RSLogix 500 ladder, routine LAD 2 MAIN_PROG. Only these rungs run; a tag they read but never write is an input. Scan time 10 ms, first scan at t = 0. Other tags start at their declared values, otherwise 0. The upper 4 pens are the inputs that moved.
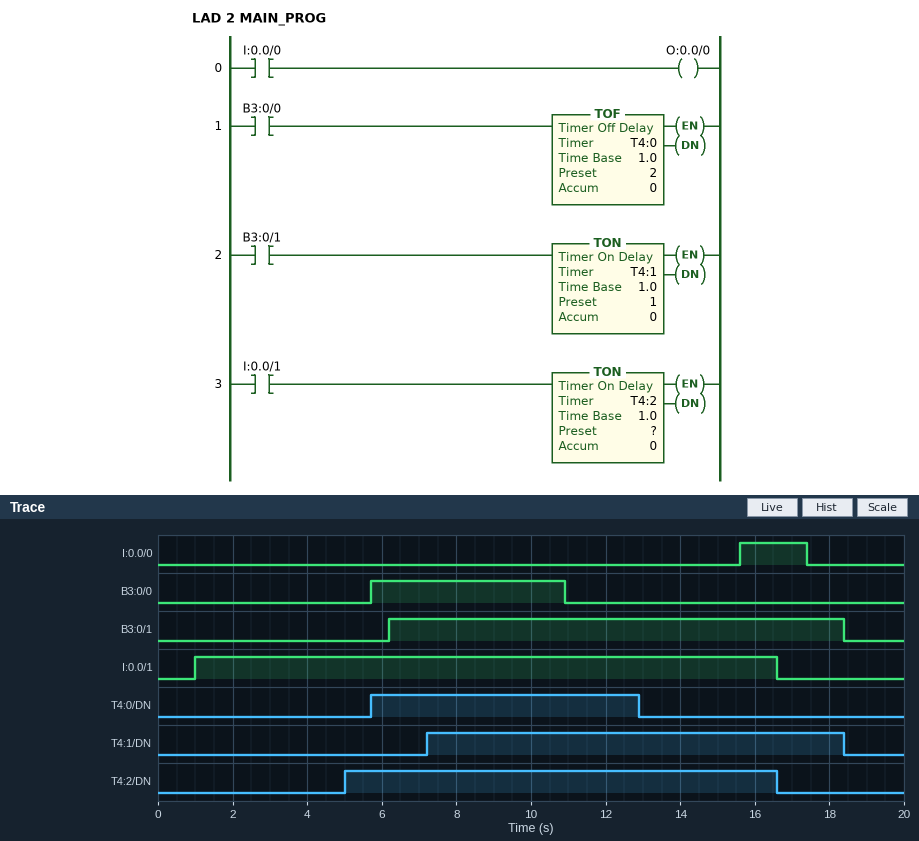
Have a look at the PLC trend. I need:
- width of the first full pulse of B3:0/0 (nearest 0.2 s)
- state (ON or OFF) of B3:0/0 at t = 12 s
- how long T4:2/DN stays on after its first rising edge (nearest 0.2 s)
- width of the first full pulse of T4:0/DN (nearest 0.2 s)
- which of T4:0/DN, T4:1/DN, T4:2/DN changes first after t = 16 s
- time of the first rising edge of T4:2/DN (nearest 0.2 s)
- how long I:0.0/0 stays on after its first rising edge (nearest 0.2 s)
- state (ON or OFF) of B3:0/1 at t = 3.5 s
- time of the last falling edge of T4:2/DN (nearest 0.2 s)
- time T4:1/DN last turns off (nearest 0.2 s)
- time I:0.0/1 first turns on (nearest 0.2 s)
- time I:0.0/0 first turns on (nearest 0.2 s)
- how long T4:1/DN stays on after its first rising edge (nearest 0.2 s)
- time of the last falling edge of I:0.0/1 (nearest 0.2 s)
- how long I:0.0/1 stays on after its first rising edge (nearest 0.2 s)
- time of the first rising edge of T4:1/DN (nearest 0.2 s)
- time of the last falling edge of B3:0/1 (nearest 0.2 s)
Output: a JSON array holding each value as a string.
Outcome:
["5.2 s", "OFF", "11.6 s", "7.2 s", "T4:2/DN", "5.0 s", "1.8 s", "OFF", "16.6 s", "18.4 s", "1.0 s", "15.6 s", "11.2 s", "16.6 s", "15.6 s", "7.2 s", "18.4 s"]
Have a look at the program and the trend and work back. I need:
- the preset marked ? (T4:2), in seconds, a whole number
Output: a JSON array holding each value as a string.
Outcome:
["4 s"]
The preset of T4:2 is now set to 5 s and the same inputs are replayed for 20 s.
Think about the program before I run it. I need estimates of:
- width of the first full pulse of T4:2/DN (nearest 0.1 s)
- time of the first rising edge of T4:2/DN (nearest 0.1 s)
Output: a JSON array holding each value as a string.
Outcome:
["10.6 s", "6.0 s"]
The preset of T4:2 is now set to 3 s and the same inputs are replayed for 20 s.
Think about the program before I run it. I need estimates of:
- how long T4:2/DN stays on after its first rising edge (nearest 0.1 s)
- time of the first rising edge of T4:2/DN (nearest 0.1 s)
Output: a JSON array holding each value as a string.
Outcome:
["12.6 s", "4.0 s"]
